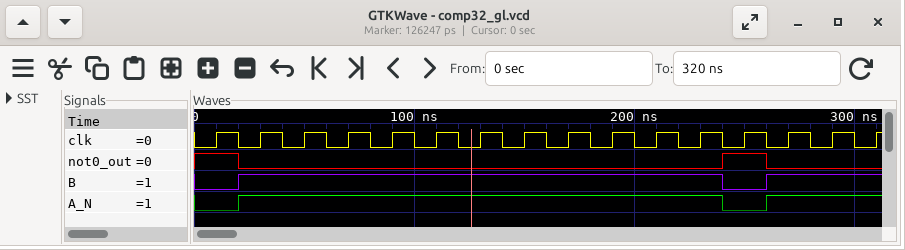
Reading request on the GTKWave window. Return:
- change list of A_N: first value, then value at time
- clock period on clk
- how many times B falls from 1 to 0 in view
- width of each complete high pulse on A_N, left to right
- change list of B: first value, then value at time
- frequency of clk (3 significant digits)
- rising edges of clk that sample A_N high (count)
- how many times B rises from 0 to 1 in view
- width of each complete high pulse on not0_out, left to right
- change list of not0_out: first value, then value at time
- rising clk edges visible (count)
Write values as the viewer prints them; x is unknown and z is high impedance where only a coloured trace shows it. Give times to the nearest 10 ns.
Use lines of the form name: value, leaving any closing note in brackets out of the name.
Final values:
change list of A_N: first value, then value at time: 0, 1 at 20 ns, 0 at 240 ns, 1 at 260 ns
clock period on clk: 20 ns
how many times B falls from 1 to 0 in view: 1
width of each complete high pulse on A_N, left to right: 220 ns
change list of B: first value, then value at time: 0, 1 at 20 ns, 0 at 240 ns, 1 at 260 ns
frequency of clk: 50.0 MHz
rising edges of clk that sample A_N high: 14
how many times B rises from 0 to 1 in view: 2
width of each complete high pulse on not0_out, left to right: 20 ns
change list of not0_out: first value, then value at time: 1, 0 at 20 ns, 1 at 240 ns, 0 at 260 ns
rising clk edges visible: 16
